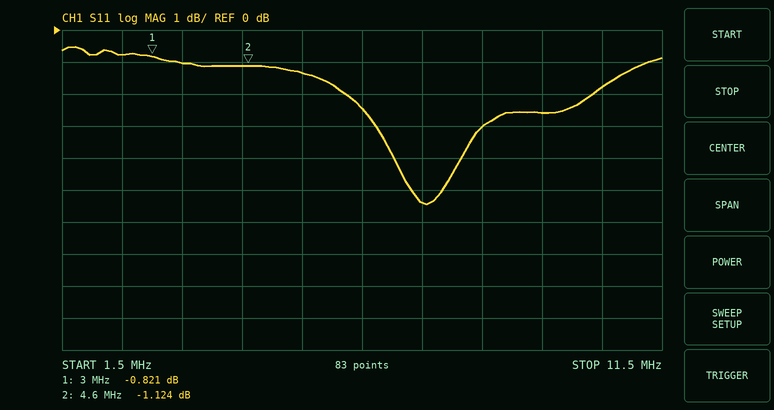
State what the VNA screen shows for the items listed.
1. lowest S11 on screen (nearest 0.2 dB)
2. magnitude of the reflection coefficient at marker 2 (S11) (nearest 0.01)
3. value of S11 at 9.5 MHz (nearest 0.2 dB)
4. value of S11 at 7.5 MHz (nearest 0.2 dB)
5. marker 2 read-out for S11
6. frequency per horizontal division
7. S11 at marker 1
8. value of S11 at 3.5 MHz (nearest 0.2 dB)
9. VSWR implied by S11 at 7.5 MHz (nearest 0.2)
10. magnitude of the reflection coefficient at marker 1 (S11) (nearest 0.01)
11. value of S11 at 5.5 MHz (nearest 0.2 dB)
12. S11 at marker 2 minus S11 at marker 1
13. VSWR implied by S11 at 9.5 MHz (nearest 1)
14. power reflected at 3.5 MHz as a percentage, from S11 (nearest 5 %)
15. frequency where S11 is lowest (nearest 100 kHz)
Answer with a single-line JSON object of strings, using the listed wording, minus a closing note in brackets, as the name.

{"lowest S11 on screen": "-5.4 dB", "magnitude of the reflection coefficient at marker 2 (S11)": "0.88", "value of S11 at 9.5 MHz": "-2.6 dB", "value of S11 at 7.5 MHz": "-5.4 dB", "marker 2 read-out for S11": "-1.124 dB", "frequency per horizontal division": "1 MHz", "S11 at marker 1": "-0.821 dB", "value of S11 at 3.5 MHz": "-1.0 dB", "VSWR implied by S11 at 7.5 MHz": "3.4", "magnitude of the reflection coefficient at marker 1 (S11)": "0.91", "value of S11 at 5.5 MHz": "-1.4 dB", "S11 at marker 2 minus S11 at marker 1": "-0.303 dB", "VSWR implied by S11 at 9.5 MHz": "7", "power reflected at 3.5 MHz as a percentage, from S11": "80 %", "frequency where S11 is lowest": "7.6 MHz"}
